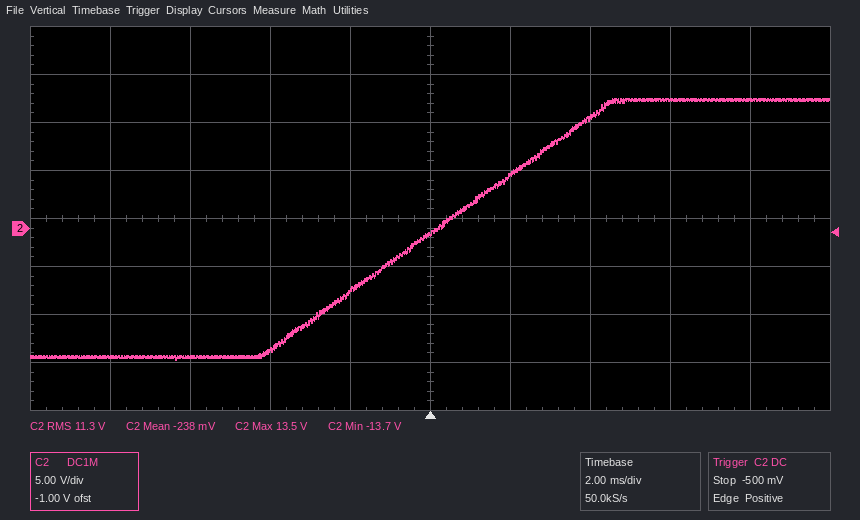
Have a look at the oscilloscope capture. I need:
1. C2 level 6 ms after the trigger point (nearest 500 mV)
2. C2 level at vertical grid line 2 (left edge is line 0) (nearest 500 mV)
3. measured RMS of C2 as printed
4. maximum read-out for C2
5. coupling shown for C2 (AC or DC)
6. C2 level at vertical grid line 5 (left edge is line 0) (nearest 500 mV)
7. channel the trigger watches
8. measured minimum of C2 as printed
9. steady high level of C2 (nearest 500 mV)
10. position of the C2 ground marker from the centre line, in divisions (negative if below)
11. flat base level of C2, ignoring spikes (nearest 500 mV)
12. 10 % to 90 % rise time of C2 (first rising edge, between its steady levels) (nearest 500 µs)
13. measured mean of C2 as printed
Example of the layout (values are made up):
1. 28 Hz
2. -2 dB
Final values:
1. 13.5 V
2. -13.5 V
3. 11.3 V
4. 13.5 V
5. DC
6. -500 mV
7. C2
8. -13.7 V
9. 13.5 V
10. -0.2 div
11. -13.5 V
12. 7.0 ms
13. -238 mV
